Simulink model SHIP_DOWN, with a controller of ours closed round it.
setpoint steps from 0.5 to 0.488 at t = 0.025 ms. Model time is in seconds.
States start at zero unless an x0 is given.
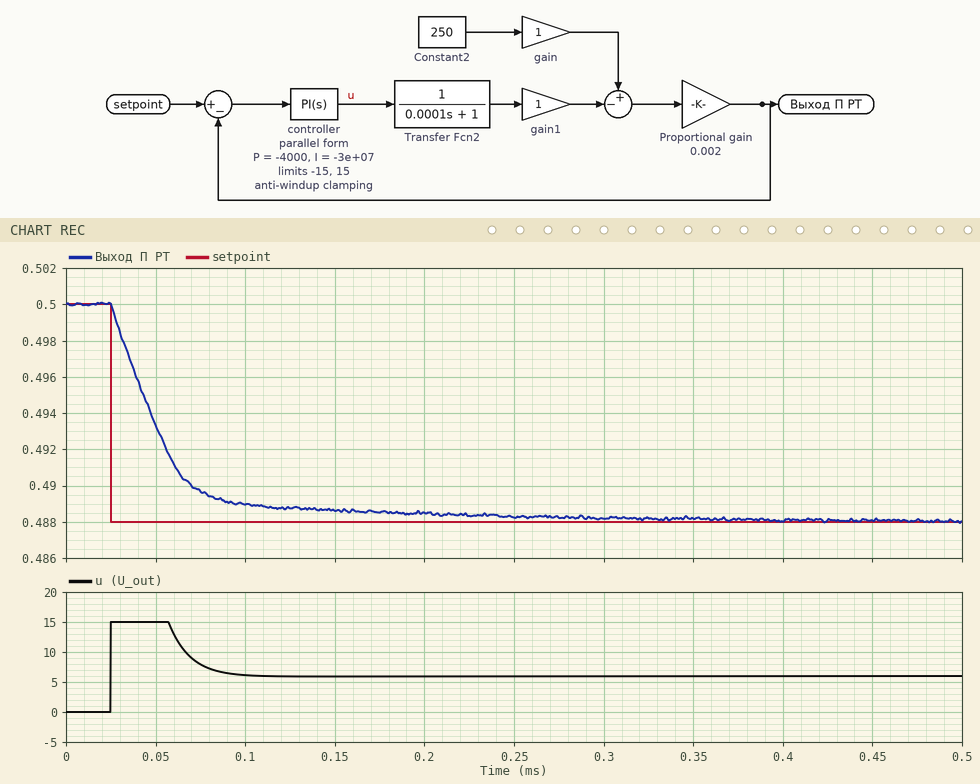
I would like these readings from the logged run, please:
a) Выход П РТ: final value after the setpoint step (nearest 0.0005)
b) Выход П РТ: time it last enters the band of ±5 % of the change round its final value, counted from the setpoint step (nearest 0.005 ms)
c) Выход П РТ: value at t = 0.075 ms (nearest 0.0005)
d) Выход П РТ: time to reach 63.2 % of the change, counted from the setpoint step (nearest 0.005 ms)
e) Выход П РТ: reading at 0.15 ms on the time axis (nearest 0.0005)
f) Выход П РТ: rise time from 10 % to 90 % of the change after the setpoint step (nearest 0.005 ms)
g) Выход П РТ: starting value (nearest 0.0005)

0.4880
0.130 ms
0.4895
0.030 ms
0.4885
0.060 ms
0.5000
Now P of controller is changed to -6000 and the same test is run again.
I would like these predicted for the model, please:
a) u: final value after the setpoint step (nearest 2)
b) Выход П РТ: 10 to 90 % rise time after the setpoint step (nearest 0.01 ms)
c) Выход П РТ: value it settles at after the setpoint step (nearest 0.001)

6
0.05 ms
0.488
